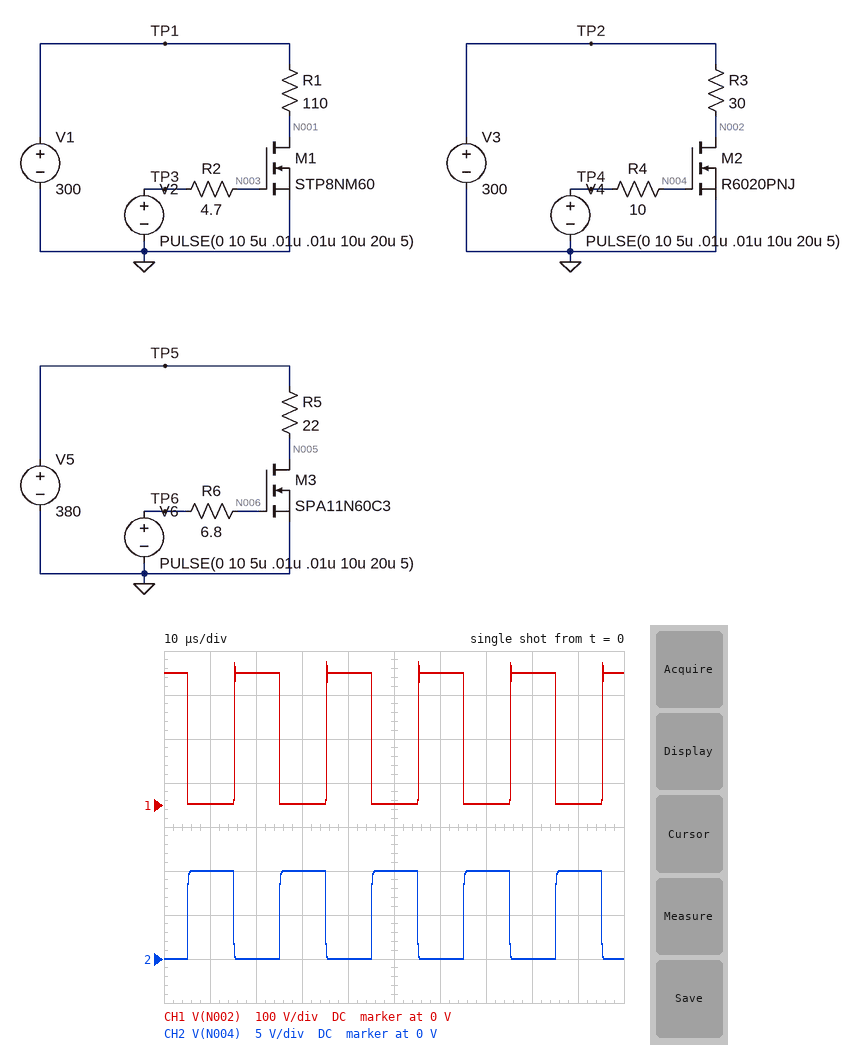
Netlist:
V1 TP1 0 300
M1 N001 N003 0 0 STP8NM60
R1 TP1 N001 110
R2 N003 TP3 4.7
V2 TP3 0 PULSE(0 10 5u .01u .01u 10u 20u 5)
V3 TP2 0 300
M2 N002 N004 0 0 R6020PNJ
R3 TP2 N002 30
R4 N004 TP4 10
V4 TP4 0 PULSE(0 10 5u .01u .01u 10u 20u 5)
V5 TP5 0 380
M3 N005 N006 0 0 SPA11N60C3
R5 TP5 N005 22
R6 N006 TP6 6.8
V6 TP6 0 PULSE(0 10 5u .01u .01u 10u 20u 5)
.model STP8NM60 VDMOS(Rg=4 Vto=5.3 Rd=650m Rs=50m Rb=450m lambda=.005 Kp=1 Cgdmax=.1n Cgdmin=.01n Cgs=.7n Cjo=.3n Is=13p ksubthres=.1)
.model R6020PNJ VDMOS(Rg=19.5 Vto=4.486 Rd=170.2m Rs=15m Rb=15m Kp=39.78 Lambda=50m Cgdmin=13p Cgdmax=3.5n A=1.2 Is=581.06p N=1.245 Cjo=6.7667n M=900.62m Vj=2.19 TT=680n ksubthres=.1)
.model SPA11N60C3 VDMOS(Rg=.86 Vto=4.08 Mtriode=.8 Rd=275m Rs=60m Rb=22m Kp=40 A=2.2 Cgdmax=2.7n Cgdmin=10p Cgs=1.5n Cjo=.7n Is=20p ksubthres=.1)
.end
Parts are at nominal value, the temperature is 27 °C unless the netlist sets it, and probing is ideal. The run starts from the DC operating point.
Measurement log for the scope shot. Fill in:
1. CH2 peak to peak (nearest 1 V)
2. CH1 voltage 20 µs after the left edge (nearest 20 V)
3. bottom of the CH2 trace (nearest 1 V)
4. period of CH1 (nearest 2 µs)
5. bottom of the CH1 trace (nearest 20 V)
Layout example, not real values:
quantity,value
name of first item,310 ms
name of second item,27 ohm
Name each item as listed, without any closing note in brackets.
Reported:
quantity,value
CH2 peak to peak,10 V
CH1 voltage 20 µs after the left edge,300 V
bottom of the CH2 trace,0 V
period of CH1,20 µs
bottom of the CH1 trace,0 V
